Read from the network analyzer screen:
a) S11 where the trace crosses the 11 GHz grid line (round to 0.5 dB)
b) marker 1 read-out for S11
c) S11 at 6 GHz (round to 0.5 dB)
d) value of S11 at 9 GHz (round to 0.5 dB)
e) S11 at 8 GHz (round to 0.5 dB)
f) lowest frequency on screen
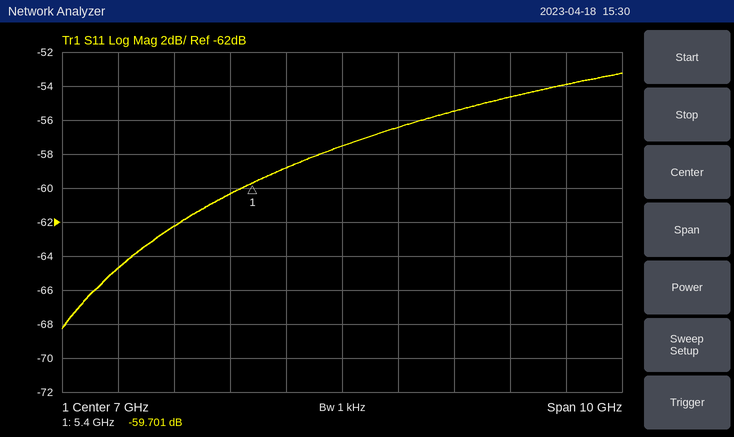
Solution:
-54.0 dB
-59.701 dB
-59.0 dB
-55.5 dB
-56.5 dB
2 GHz
